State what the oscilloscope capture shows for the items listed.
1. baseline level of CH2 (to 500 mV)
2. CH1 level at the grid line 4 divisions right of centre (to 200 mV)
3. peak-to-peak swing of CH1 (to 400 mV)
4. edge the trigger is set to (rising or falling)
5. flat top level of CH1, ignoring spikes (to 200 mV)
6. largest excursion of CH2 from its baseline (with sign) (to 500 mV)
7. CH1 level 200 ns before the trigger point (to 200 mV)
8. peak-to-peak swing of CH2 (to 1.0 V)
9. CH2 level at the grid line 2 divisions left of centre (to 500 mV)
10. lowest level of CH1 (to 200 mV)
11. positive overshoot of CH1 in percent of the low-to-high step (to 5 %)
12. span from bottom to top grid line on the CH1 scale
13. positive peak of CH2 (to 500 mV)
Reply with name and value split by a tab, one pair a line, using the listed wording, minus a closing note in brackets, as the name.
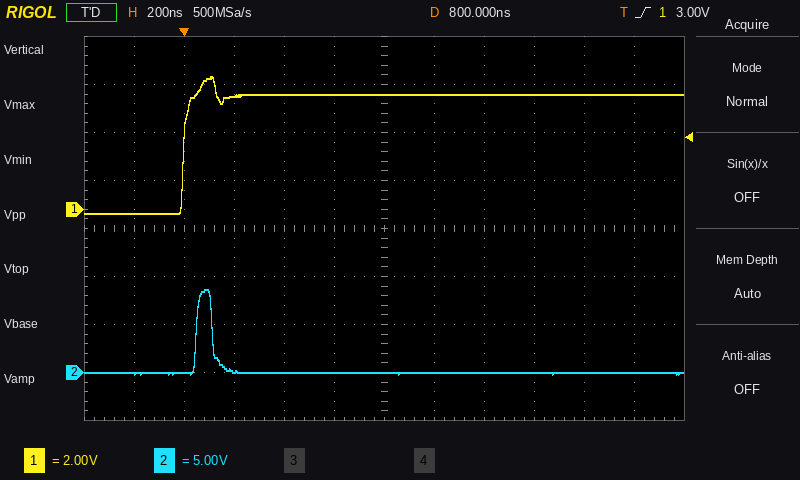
baseline level of CH2	0.0 V
CH1 level at the grid line 4 divisions right of centre	4.8 V
peak-to-peak swing of CH1	5.6 V
edge the trigger is set to	rising
flat top level of CH1, ignoring spikes	4.8 V
largest excursion of CH2 from its baseline (with sign)	+8.5 V
CH1 level 200 ns before the trigger point	-200 mV
peak-to-peak swing of CH2	9.0 V
CH2 level at the grid line 2 divisions left of centre	0.0 V
lowest level of CH1	-200 mV
positive overshoot of CH1 in percent of the low-to-high step	15 %
span from bottom to top grid line on the CH1 scale	16 V
positive peak of CH2	8.5 V
